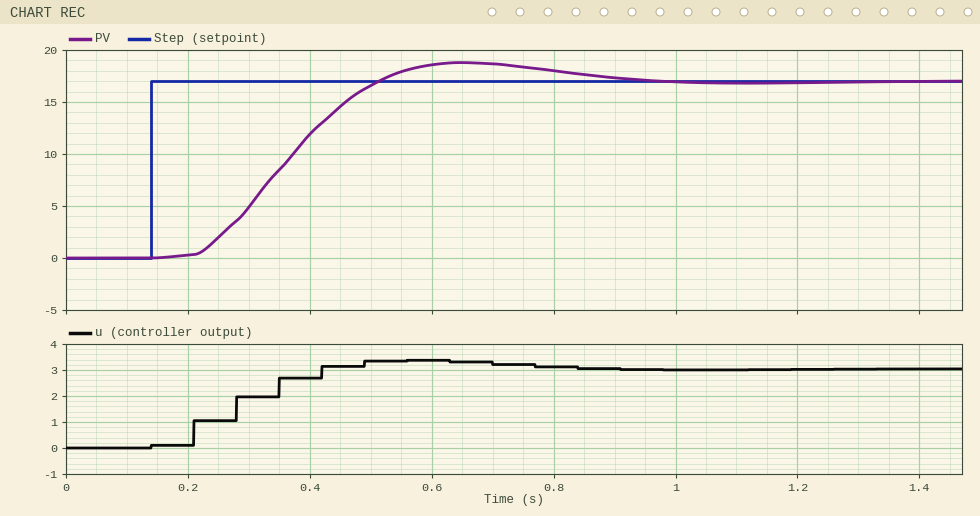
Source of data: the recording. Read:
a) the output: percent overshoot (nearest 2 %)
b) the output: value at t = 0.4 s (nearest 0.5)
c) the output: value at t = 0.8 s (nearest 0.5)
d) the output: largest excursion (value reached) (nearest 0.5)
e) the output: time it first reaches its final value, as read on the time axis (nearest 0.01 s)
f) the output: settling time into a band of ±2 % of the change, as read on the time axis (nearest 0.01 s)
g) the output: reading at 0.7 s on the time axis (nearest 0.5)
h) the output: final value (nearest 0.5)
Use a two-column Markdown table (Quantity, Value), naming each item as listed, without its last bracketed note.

| Quantity | Value |
|---|---|
| the output: percent overshoot | 10 % |
| the output: value at t = 0.4 s | 12.0 |
| the output: value at t = 0.8 s | 18.0 |
| the output: largest excursion (value reached) | 19.0 |
| the output: time it first reaches its final value, as read on the time axis | 0.51 s |
| the output: settling time into a band of ±2 % of the change, as read on the time axis | 0.90 s |
| the output: reading at 0.7 s on the time axis | 18.5 |
| the output: final value | 17.0 |
